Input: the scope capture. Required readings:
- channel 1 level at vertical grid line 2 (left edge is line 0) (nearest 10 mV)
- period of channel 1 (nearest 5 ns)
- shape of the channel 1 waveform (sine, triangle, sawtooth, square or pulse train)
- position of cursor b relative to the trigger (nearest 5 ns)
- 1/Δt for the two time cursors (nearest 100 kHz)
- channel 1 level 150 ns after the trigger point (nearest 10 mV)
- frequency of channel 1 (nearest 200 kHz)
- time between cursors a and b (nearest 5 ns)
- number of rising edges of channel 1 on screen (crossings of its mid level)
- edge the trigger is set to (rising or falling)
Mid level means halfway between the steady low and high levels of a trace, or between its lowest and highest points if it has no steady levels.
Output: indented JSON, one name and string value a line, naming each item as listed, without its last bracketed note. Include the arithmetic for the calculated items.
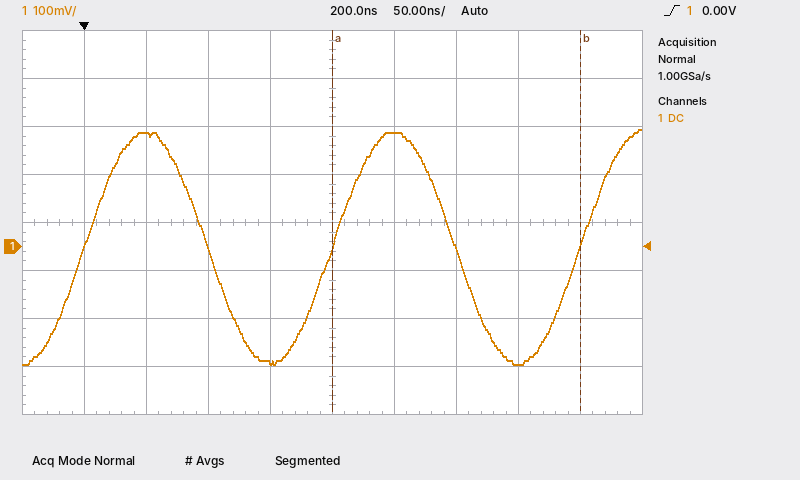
{
  "channel 1 level at vertical grid line 2 (left edge is line 0)": "240 mV",
  "period of channel 1": "200 ns",
  "shape of the channel 1 waveform": "sine",
  "position of cursor b relative to the trigger": "+400 ns",
  "1/Δt for the two time cursors": "1 / 200 ns ≈ 5.0 MHz",
  "channel 1 level 150 ns after the trigger point": "-240 mV",
  "frequency of channel 1": "1 / 200 ns ≈ 5.0 MHz",
  "time between cursors a and b": "200 ns",
  "number of rising edges of channel 1 on screen": "3",
  "edge the trigger is set to": "rising"
}
